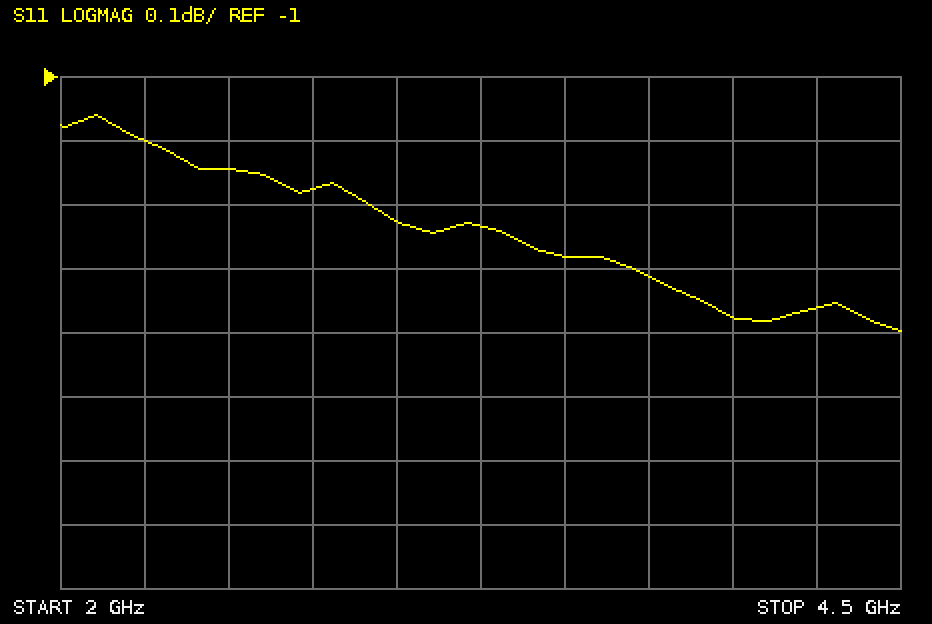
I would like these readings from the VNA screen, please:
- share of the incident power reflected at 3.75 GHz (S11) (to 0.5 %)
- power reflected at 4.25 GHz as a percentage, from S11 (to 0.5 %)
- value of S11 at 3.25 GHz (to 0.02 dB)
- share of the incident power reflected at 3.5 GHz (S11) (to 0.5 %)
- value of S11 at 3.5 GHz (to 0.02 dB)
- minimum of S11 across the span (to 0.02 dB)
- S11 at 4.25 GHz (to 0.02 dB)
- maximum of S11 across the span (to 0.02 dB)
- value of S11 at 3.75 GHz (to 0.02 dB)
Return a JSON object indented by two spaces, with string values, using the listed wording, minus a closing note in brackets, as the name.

{
  "share of the incident power reflected at 3.75 GHz (S11)": "74.0 %",
  "power reflected at 4.25 GHz as a percentage, from S11": "73.0 %",
  "value of S11 at 3.25 GHz": "-1.24 dB",
  "share of the incident power reflected at 3.5 GHz (S11)": "74.5 %",
  "value of S11 at 3.5 GHz": "-1.28 dB",
  "minimum of S11 across the span": "-1.40 dB",
  "S11 at 4.25 GHz": "-1.36 dB",
  "maximum of S11 across the span": "-1.06 dB",
  "value of S11 at 3.75 GHz": "-1.32 dB"
}
